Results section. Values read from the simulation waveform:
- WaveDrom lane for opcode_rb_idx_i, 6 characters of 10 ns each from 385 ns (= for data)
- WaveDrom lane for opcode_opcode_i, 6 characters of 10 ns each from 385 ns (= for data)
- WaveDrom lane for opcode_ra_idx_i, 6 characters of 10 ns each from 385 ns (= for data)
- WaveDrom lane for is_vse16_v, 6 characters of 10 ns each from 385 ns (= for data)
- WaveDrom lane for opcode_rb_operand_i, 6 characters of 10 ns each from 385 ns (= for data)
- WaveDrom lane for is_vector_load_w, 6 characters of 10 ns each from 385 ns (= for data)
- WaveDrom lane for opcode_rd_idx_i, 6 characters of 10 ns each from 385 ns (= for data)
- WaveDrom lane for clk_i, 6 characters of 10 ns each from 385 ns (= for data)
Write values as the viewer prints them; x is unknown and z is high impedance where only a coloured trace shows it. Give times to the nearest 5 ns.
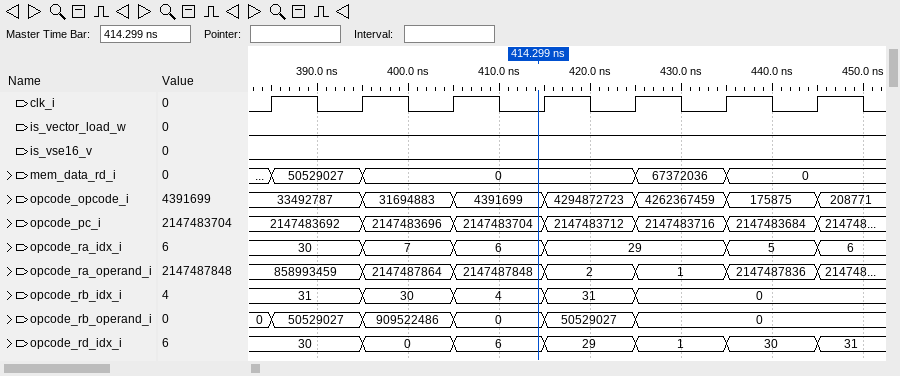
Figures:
{name: 'opcode_rb_idx_i', wave: '=====.', data: '31 30 4 31 0'}
{name: 'opcode_opcode_i', wave: '======', data: '33492787 31694883 4391699 4294872723 4262367459 175875'}
{name: 'opcode_ra_idx_i', wave: '====.=', data: '30 7 6 29 5'}
{name: 'is_vse16_v', wave: '0.....'}
{name: 'opcode_rb_operand_i', wave: '=====.', data: '50529027 909522486 0 50529027 0'}
{name: 'is_vector_load_w', wave: '0.....'}
{name: 'opcode_rd_idx_i', wave: '======', data: '30 0 6 29 1 30'}
{name: 'clk_i', wave: 'p.....'}
